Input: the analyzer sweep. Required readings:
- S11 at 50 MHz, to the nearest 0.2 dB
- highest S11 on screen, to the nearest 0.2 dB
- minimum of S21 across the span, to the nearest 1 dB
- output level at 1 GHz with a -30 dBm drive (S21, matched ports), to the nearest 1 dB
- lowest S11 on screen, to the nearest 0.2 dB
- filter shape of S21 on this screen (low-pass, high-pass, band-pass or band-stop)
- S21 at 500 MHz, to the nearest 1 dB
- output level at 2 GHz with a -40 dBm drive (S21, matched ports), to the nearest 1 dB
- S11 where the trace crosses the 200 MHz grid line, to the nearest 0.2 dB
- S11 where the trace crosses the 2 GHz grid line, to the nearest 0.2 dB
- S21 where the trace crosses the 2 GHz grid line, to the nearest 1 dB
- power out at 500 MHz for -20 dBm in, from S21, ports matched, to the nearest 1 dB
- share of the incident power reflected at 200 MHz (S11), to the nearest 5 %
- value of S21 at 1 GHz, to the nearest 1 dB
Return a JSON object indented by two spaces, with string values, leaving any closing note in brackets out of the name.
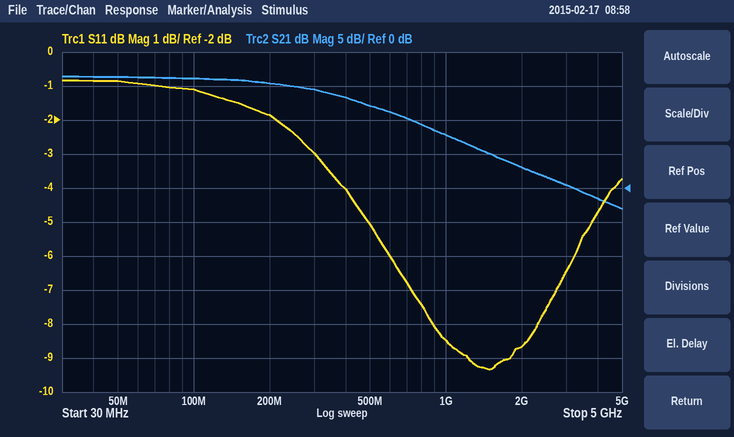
{
  "S11 at 50 MHz, to the nearest 0.2 dB": "-0.8 dB",
  "highest S11 on screen, to the nearest 0.2 dB": "-0.8 dB",
  "minimum of S21 across the span, to the nearest 1 dB": "-3 dB",
  "output level at 1 GHz with a -30 dBm drive (S21, matched ports), to the nearest 1 dB": "-22 dBm",
  "lowest S11 on screen, to the nearest 0.2 dB": "-9.4 dB",
  "filter shape of S21 on this screen": "low-pass",
  "S21 at 500 MHz, to the nearest 1 dB": "12 dB",
  "output level at 2 GHz with a -40 dBm drive (S21, matched ports), to the nearest 1 dB": "-37 dBm",
  "S11 where the trace crosses the 200 MHz grid line, to the nearest 0.2 dB": "-1.8 dB",
  "S11 where the trace crosses the 2 GHz grid line, to the nearest 0.2 dB": "-8.6 dB",
  "S21 where the trace crosses the 2 GHz grid line, to the nearest 1 dB": "3 dB",
  "power out at 500 MHz for -20 dBm in, from S21, ports matched, to the nearest 1 dB": "-8 dBm",
  "share of the incident power reflected at 200 MHz (S11), to the nearest 5 %": "65 %",
  "value of S21 at 1 GHz, to the nearest 1 dB": "8 dB"
}
